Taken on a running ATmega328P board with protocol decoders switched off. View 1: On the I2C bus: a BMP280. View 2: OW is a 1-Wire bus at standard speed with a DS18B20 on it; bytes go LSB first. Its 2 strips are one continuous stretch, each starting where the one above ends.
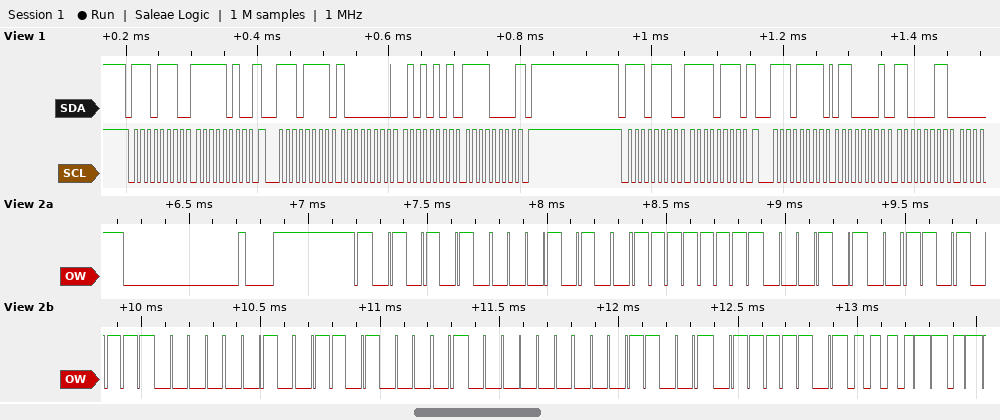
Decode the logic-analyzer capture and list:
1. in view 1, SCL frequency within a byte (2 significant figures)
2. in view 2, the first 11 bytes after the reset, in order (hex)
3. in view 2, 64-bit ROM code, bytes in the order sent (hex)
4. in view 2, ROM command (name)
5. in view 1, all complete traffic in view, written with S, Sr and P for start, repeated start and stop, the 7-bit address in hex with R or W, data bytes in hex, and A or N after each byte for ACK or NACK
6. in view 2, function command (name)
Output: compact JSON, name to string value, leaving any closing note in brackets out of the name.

{"in view 1, SCL frequency within a byte": "100 kHz", "in view 2, the first 11 bytes after the reset, in order": "55 28 FF 28 EB 40 16 02 98 BE B0", "in view 2, 64-bit ROM code, bytes in the order sent": "28 FF 28 EB 40 16 02 98", "in view 2, ROM command": "Match ROM", "in view 1, all complete traffic in view, written with S, Sr and P for start, repeated start and stop, the 7-bit address in hex with R or W, data bytes in hex, and A or N after each byte for ACK or NACK": "S 77W A FA A Sr 77R A 80 A 55 A F0 N P S 77W A F7 A Sr 77R A 61 A C3 A", "in view 2, function command": "Read Scratchpad"}
